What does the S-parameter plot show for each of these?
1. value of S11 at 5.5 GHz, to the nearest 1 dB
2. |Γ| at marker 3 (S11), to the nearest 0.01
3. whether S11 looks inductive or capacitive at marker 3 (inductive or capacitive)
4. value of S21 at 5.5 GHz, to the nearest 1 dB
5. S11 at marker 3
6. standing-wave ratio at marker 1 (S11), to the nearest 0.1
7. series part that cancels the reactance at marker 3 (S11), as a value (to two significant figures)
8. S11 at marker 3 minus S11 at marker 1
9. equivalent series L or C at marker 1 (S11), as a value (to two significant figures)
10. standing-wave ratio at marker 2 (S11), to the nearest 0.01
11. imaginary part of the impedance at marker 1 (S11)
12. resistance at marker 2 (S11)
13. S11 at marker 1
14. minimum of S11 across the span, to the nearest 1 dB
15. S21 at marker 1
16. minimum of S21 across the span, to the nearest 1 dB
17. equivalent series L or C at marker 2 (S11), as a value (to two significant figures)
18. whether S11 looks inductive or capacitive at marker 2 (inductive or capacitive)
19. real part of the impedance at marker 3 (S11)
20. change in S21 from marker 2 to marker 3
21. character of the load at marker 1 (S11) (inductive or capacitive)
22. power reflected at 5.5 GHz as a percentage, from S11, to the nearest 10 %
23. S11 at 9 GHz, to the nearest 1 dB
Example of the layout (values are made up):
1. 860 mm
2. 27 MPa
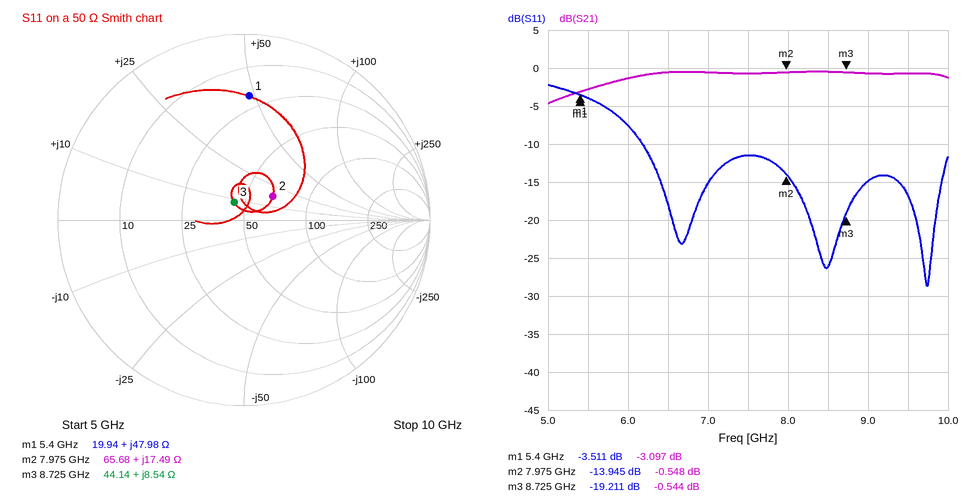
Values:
1. -4 dB
2. 0.11
3. inductive
4. -3 dB
5. -19.211 dB
6. 5.0
7. 2.1 pF
8. -15.700 dB
9. 1.4 nH
10. 1.50
11. +47.98 Ω
12. 65.68 Ω
13. -3.511 dB
14. -29 dB
15. -3.097 dB
16. -5 dB
17. 350 pH
18. inductive
19. 44.14 Ω
20. 0.004 dB
21. inductive
22. 40 %
23. -15 dB
